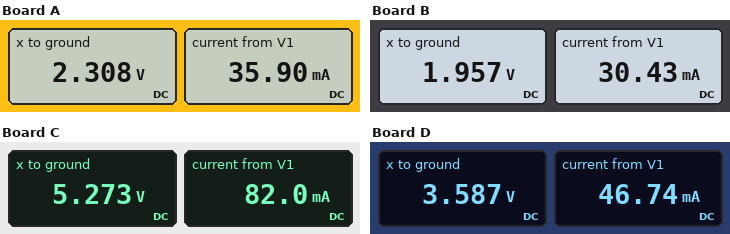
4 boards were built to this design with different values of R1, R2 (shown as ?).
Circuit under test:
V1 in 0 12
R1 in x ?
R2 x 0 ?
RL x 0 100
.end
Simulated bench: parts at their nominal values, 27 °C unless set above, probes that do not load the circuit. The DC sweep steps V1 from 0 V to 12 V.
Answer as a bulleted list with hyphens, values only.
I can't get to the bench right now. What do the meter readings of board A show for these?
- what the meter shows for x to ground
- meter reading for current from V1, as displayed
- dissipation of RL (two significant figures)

- 2.308 V
- 35.90 mA
- 53 mW
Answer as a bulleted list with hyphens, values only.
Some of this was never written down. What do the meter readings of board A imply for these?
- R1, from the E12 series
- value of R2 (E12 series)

- 270 Ω
- 180 Ω
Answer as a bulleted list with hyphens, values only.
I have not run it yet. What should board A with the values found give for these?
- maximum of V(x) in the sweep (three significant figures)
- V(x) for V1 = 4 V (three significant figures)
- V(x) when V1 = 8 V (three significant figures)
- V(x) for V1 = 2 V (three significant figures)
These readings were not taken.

- 2.31 V
- 769 mV
- 1.54 V
- 385 mV
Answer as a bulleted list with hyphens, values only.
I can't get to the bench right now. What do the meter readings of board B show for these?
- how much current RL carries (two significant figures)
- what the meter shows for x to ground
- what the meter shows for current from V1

- 20 mA
- 1.957 V
- 30.43 mA
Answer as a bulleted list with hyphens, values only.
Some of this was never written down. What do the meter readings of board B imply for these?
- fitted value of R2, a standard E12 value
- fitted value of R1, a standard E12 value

- 180 Ω
- 330 Ω
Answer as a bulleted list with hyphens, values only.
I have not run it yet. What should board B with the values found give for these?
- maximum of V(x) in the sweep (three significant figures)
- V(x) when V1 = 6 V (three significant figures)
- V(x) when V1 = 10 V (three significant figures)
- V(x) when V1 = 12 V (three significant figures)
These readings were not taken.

- 1.96 V
- 978 mV
- 1.63 V
- 1.96 V
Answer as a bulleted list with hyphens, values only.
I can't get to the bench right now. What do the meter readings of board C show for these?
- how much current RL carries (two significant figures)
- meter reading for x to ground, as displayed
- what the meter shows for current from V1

- 53 mA
- 5.273 V
- 82.0 mA
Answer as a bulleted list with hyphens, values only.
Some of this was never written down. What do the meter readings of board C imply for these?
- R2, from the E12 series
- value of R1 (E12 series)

- 180 Ω
- 82 Ω
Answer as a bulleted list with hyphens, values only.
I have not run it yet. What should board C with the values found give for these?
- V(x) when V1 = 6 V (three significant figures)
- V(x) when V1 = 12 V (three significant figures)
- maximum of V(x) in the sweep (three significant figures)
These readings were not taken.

- 2.64 V
- 5.27 V
- 5.27 V
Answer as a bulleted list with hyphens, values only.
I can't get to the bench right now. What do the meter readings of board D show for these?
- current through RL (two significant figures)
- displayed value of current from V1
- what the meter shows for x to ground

- 36 mA
- 46.74 mA
- 3.587 V
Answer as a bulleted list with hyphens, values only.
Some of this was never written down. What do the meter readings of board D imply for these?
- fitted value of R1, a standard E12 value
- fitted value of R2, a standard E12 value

- 180 Ω
- 330 Ω
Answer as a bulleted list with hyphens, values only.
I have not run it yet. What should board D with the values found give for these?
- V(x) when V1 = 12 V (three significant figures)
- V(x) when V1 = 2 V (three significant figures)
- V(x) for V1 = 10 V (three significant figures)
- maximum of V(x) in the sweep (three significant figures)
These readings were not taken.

- 3.59 V
- 598 mV
- 2.99 V
- 3.59 V
